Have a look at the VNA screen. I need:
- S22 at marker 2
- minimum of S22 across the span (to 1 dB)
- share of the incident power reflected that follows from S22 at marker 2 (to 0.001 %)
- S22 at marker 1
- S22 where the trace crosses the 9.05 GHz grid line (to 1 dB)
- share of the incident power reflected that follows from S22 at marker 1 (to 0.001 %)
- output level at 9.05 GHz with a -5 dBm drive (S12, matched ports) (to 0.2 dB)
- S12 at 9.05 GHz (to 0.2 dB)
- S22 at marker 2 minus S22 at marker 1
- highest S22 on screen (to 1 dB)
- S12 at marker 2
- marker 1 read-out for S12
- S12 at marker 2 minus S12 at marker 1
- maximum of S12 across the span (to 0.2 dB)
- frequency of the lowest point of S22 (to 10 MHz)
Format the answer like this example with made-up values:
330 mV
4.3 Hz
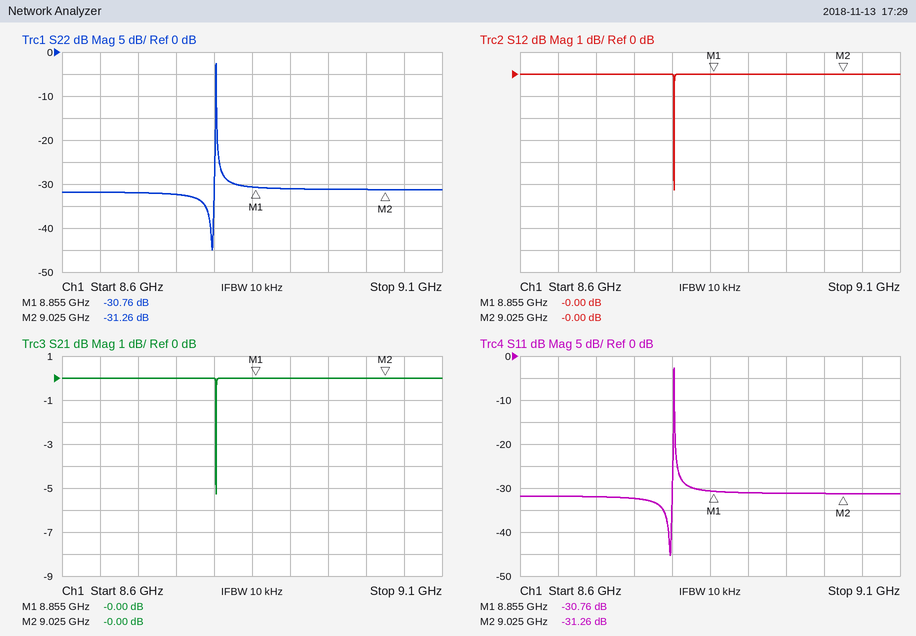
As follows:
-31.26 dB
-45 dB
0.075 %
-30.76 dB
-31 dB
0.084 %
-5.0 dBm
0.0 dB
-0.50 dB
-3 dB
-0.00 dB
-0.00 dB
0.00 dB
0.0 dB
8.80 GHz
